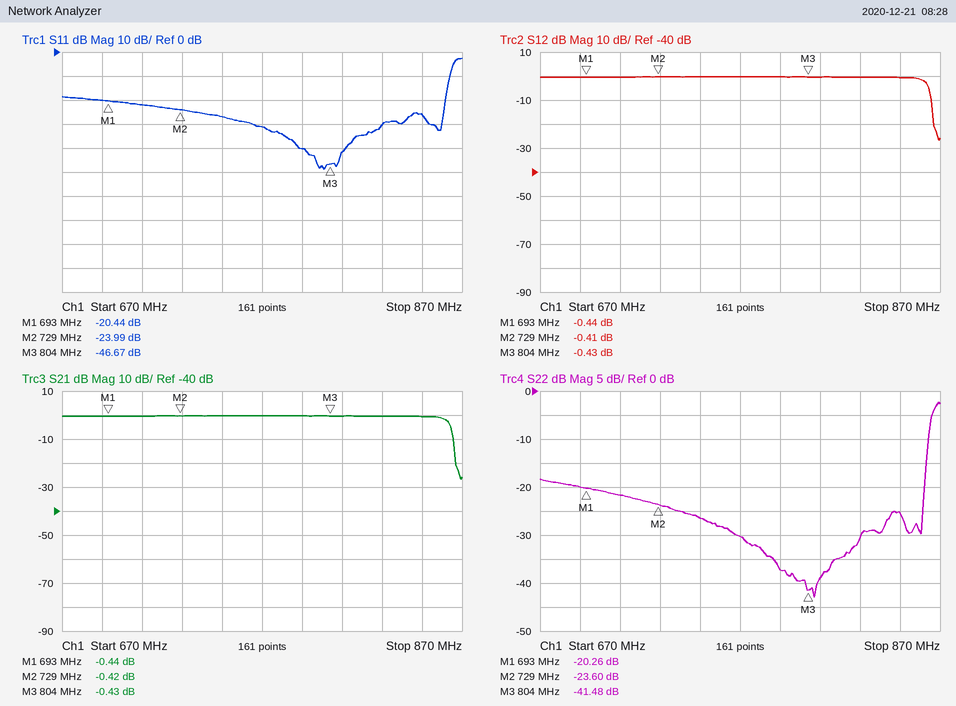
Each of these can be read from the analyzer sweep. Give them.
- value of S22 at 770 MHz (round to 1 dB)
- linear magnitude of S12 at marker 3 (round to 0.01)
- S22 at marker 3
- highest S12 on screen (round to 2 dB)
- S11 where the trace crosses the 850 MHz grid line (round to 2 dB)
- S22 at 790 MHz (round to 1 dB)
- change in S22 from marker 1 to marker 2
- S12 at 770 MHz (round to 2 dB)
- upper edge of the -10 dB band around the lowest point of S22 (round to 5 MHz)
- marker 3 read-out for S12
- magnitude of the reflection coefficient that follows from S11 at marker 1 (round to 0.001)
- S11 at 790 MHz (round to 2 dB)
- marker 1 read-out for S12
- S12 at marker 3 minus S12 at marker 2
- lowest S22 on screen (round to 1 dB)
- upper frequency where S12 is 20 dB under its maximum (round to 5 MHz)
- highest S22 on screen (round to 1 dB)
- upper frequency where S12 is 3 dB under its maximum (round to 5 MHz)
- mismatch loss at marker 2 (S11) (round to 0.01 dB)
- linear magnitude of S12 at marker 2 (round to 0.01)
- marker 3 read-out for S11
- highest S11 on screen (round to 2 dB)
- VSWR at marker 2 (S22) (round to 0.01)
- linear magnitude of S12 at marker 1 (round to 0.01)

-30 dB
0.95
-41.48 dB
0 dB
-26 dB
-37 dB
-3.34 dB
0 dB
865 MHz
-0.43 dB
0.095
-40 dB
-0.44 dB
-0.02 dB
-43 dB
865 MHz
-2 dB
865 MHz
0.02 dB
0.95
-46.67 dB
-2 dB
1.14
0.95
